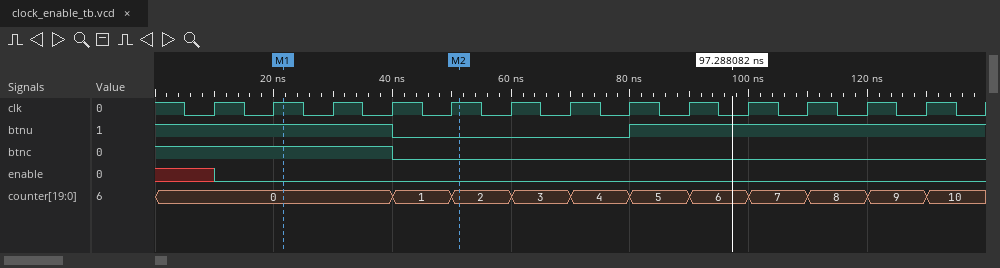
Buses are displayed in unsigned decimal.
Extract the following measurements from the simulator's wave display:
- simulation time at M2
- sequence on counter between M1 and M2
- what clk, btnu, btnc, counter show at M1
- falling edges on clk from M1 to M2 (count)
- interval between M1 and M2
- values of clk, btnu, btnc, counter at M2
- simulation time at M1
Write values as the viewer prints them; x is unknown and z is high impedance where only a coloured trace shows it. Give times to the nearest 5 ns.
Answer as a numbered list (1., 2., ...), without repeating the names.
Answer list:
1. 50 ns
2. 0, 1, 2
3. clk=1, btnu=1, btnc=1, counter=0
4. 3
5. 30 ns
6. clk=1, btnu=0, btnc=0, counter=2
7. 20 ns
